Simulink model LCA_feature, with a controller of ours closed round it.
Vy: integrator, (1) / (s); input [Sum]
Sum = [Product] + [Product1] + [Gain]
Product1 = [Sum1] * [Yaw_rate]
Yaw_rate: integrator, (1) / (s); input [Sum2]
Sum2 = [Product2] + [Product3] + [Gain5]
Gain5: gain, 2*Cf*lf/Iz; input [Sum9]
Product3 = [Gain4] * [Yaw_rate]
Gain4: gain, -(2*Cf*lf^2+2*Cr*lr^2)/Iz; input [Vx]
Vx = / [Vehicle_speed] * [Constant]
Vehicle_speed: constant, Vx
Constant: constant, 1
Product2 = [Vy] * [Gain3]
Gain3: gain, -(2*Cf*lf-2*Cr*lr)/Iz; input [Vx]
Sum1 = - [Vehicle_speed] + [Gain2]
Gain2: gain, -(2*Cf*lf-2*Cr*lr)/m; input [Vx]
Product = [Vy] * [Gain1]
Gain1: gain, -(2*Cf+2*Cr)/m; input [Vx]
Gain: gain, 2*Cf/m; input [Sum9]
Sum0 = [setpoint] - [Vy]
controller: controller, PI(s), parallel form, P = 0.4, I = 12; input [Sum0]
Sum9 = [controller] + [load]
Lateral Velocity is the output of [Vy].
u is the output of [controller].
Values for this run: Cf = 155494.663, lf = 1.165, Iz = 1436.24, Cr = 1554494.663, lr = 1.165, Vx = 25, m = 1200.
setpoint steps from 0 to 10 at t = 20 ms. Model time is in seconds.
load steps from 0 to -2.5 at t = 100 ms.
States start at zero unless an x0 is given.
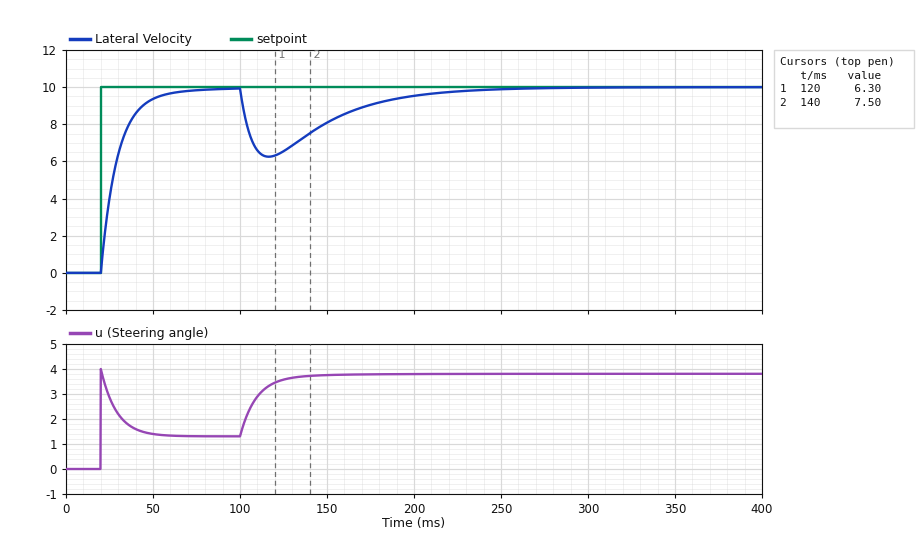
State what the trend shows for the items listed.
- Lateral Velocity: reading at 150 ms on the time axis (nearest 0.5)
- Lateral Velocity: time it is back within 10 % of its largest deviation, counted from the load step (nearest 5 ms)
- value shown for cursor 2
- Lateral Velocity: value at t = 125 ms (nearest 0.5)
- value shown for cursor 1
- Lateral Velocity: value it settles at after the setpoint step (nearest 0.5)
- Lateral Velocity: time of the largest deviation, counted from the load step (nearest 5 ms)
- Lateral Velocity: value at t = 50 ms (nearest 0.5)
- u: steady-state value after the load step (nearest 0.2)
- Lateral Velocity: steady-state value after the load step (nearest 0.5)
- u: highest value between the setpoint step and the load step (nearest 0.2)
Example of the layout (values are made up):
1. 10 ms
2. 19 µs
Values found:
1. 8.0
2. 110 ms
3. 7.50
4. 6.5
5. 6.30
6. 10.0
7. 15 ms
8. 9.5
9. 3.8
10. 10.0
11. 4.0
